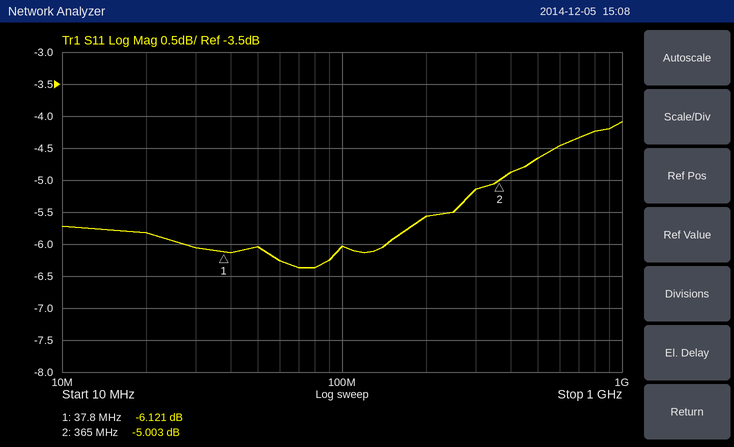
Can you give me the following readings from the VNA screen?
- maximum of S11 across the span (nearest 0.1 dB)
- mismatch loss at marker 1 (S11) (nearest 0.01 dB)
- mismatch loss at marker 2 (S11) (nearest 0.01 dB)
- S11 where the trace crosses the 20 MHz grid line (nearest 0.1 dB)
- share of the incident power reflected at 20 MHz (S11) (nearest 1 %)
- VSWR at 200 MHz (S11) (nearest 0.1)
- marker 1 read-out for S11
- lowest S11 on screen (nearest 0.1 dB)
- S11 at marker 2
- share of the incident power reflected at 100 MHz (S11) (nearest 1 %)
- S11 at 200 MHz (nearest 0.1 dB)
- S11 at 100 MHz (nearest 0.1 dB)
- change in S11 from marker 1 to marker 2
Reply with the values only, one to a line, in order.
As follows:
-4.1 dB
1.22 dB
1.65 dB
-5.8 dB
26 %
3.2
-6.121 dB
-6.4 dB
-5.003 dB
25 %
-5.6 dB
-6.0 dB
1.118 dB
